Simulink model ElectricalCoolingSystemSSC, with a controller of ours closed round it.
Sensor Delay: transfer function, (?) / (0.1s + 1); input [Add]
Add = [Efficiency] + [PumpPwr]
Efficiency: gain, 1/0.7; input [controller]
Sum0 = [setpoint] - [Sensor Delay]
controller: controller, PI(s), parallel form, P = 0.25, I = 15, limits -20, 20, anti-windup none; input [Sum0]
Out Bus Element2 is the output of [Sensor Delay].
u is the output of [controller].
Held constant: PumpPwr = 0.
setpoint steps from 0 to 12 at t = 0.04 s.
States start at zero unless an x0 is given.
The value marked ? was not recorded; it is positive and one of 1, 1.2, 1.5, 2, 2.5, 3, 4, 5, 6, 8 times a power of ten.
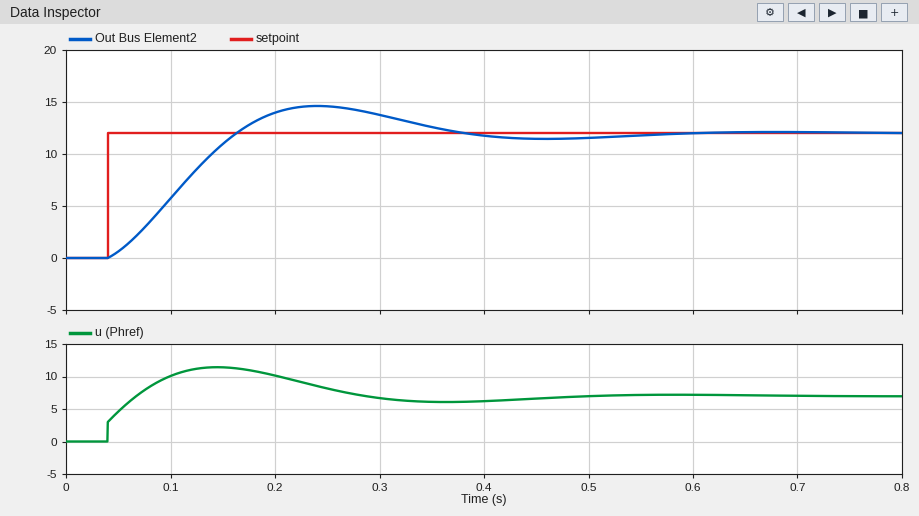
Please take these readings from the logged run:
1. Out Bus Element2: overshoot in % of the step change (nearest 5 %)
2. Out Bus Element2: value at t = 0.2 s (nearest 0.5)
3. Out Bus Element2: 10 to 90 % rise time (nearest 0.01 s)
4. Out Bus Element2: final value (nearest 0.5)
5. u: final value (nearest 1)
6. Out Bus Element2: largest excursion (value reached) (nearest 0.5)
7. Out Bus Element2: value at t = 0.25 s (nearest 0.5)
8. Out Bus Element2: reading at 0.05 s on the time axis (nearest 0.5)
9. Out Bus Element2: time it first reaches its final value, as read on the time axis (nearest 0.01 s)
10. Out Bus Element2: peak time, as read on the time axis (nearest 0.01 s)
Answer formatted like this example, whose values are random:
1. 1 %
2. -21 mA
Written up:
1. 20 %
2. 14.0
3. 0.09 s
4. 12.0
5. 7
6. 14.5
7. 14.5
8. 0.5
9. 0.16 s
10. 0.24 s
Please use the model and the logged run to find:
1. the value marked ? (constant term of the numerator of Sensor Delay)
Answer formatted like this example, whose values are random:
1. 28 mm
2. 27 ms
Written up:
1. 1.2
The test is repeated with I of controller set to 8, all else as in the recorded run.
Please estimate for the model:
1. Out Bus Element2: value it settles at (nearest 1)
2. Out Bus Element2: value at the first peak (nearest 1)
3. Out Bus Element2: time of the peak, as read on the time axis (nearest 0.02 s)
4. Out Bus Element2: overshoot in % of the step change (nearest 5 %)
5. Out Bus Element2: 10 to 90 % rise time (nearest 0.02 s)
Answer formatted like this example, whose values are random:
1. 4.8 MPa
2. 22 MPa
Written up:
1. 12
2. 13
3. 0.34 s
4. 10 %
5. 0.14 s
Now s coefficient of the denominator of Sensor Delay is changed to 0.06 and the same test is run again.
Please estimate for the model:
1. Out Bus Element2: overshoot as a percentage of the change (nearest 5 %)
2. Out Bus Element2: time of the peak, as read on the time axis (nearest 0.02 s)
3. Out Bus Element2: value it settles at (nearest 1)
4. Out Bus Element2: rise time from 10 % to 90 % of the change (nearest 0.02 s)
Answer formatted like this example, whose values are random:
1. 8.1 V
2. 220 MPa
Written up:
1. 10 %
2. 0.20 s
3. 12
4. 0.08 s
